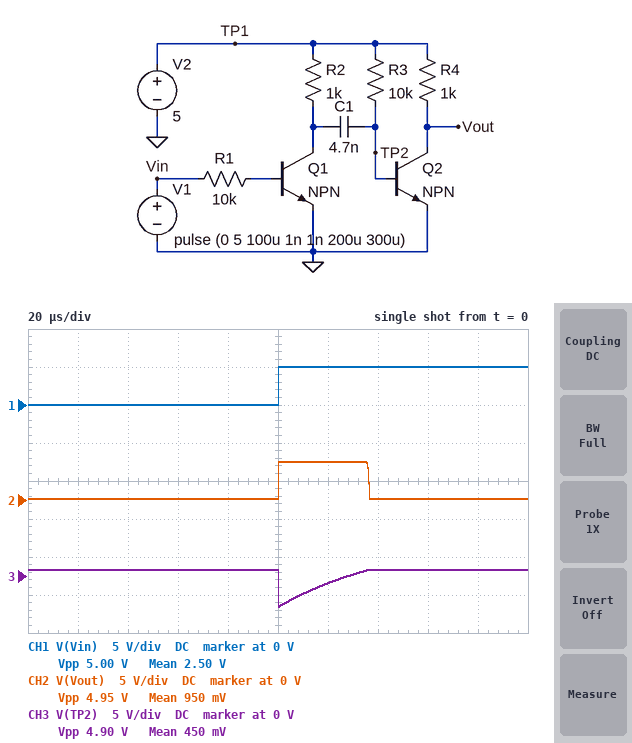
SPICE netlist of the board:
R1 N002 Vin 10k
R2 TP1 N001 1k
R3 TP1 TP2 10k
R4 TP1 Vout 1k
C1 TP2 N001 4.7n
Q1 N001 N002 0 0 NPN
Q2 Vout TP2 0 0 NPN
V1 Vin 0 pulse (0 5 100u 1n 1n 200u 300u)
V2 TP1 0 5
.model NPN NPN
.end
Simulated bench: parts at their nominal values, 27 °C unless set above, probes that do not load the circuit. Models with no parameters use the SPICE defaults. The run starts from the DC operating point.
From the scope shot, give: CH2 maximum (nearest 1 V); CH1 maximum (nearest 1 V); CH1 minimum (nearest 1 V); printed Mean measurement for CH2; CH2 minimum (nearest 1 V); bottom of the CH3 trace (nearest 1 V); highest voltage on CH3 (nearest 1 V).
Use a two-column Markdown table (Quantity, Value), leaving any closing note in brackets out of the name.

| Quantity | Value |
|---|---|
| CH2 maximum | 5 V |
| CH1 maximum | 5 V |
| CH1 minimum | 0 V |
| printed Mean measurement for CH2 | 950 mV |
| CH2 minimum | 0 V |
| bottom of the CH3 trace | -4 V |
| highest voltage on CH3 | 1 V |
